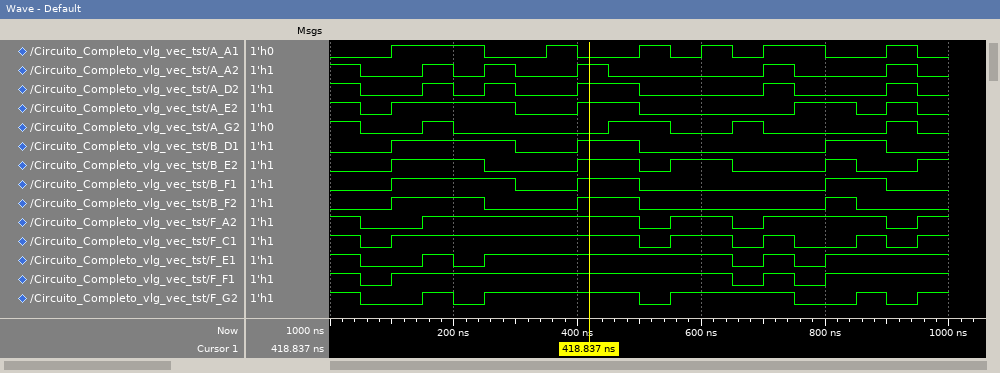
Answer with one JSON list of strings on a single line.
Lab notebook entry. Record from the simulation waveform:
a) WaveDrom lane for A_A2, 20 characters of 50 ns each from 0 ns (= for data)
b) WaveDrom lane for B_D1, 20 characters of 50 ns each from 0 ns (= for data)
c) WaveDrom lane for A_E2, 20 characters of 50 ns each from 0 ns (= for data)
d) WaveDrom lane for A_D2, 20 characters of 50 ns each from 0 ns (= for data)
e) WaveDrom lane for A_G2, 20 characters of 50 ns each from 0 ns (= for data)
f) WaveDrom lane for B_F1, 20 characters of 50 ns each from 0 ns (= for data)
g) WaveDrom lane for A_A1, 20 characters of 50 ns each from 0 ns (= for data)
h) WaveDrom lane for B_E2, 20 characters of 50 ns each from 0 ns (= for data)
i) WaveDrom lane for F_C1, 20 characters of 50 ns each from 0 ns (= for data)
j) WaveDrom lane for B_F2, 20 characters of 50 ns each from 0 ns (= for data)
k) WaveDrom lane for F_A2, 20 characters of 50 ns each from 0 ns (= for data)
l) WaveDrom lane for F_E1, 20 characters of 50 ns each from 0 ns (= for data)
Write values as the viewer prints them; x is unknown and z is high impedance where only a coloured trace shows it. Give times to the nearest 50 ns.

["{name: 'A_A2', wave: '10.1010.10....10..10'}", "{name: 'B_D1', wave: '0.1...0.1.0.....1.0.'}", "{name: 'A_E2', wave: '101...0.1.0....1.010'}", "{name: 'A_D2', wave: '10.1010.1.0...10..10'}", "{name: 'A_G2', wave: '10.10....1.0.10...10'}", "{name: 'B_F1', wave: '0.1...0.1.0.....1.0.'}", "{name: 'A_A1', wave: '0.1..0.10.10101.0.10'}", "{name: 'B_E2', wave: '0.1..0..1.01.0..10.1'}", "{name: 'F_C1', wave: '101.......01.010.101'}", "{name: 'B_F2', wave: '0.1..0..1.0.....10..'}", "{name: 'F_A2', wave: '10.1......01.01...01'}", "{name: 'F_E1', wave: '10.101.......0101...'}"]
